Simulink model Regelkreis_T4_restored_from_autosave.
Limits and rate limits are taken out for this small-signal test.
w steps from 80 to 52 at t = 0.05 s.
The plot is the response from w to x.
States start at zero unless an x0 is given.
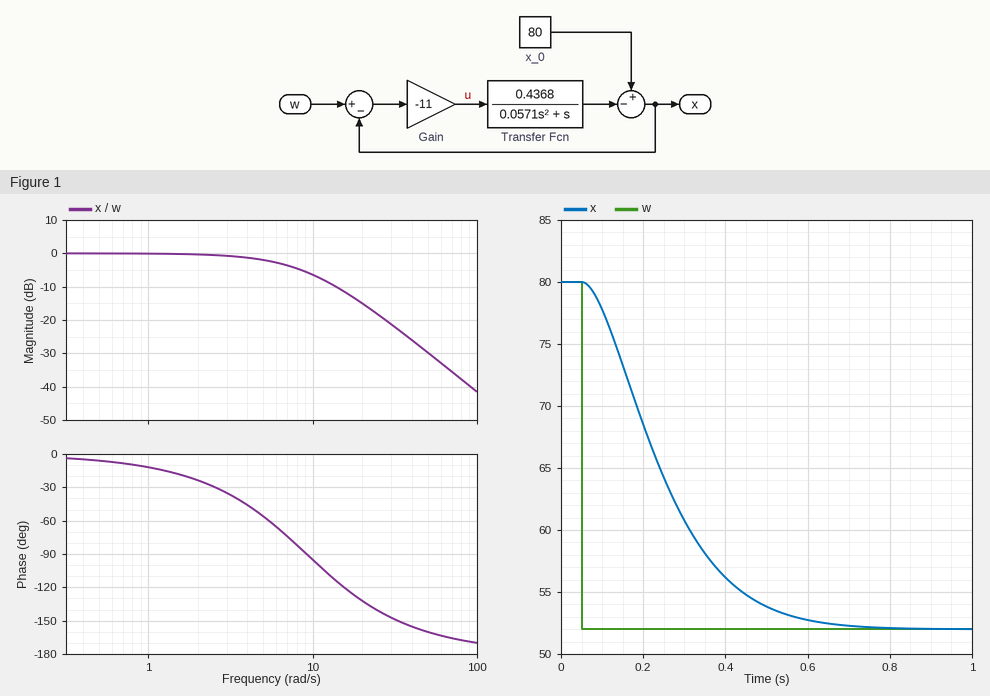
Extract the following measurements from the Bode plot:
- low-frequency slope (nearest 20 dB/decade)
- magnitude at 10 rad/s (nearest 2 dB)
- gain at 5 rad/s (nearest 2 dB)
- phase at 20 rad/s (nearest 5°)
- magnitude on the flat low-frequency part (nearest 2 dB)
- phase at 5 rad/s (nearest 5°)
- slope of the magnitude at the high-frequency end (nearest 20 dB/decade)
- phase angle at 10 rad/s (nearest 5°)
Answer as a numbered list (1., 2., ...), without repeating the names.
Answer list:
1. 0 dB/decade
2. -6 dB
3. -2 dB
4. -130°
5. 0 dB
6. -55°
7. -40 dB/decade
8. -95°
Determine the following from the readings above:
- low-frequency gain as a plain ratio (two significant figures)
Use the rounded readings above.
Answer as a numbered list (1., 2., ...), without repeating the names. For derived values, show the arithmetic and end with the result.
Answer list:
1. 10^(0 / 20) = 1.0
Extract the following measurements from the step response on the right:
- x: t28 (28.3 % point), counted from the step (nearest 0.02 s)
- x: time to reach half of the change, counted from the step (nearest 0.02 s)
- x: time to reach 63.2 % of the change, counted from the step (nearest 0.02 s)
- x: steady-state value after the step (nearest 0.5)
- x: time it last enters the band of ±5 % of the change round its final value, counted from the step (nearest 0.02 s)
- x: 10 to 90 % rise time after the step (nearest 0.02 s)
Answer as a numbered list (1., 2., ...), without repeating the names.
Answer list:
1. 0.12 s
2. 0.18 s
3. 0.22 s
4. 52.0
5. 0.48 s
6. 0.34 s
